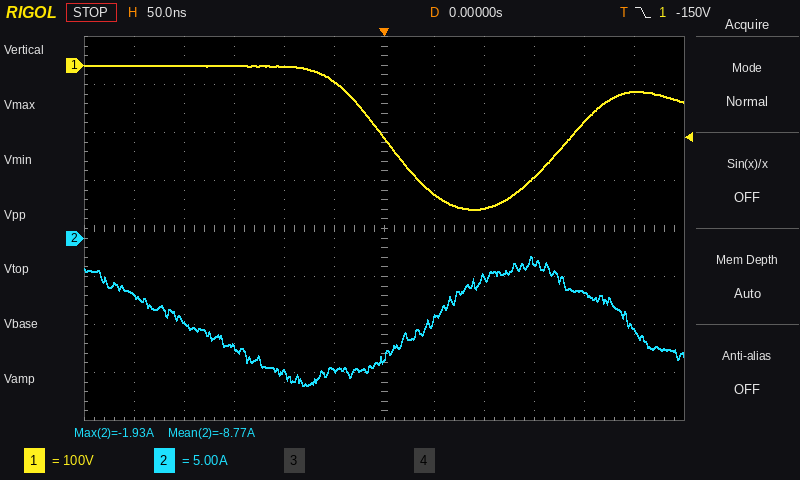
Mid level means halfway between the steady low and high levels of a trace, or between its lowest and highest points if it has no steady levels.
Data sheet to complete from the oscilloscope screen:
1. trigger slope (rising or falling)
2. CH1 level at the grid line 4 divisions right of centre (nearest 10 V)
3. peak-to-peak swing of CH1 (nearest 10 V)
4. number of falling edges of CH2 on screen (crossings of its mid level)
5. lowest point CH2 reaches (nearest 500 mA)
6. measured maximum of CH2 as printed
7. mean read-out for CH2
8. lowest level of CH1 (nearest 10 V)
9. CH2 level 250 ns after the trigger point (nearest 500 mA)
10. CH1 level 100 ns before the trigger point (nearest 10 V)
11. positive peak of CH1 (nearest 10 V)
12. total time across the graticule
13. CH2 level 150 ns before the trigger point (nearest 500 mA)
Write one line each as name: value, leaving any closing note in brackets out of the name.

trigger slope: falling
CH1 level at the grid line 4 divisions right of centre: -120 V
peak-to-peak swing of CH1: 300 V
number of falling edges of CH2 on screen: 2
lowest point CH2 reaches: -15.5 A
measured maximum of CH2 as printed: -1.93 A
mean read-out for CH2: -8.77 A
lowest level of CH1: -300 V
CH2 level 250 ns after the trigger point: -9.5 A
CH1 level 100 ns before the trigger point: 0 V
positive peak of CH1: 0 V
total time across the graticule: 600 ns
CH2 level 150 ns before the trigger point: -11.5 A
